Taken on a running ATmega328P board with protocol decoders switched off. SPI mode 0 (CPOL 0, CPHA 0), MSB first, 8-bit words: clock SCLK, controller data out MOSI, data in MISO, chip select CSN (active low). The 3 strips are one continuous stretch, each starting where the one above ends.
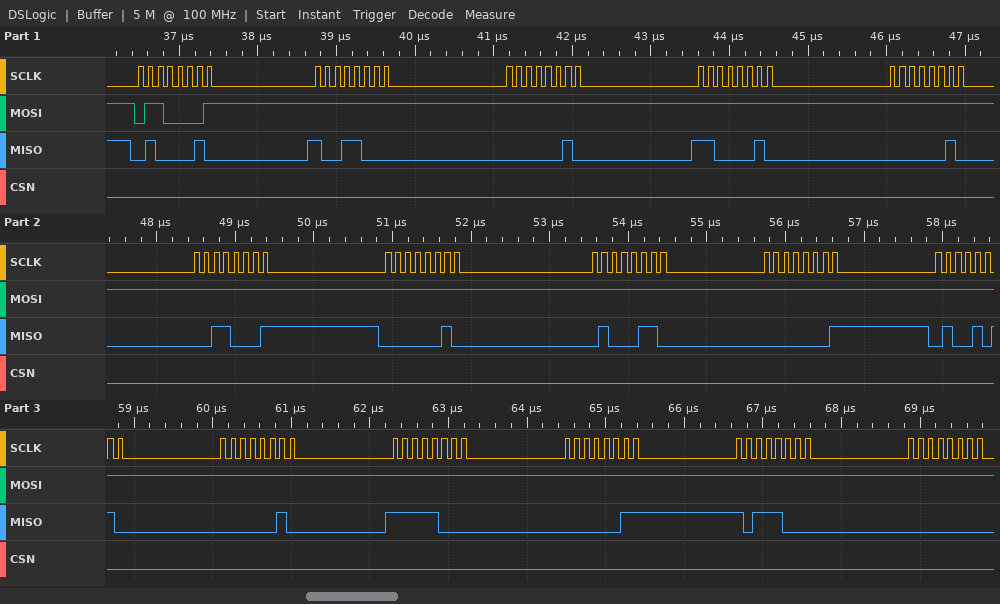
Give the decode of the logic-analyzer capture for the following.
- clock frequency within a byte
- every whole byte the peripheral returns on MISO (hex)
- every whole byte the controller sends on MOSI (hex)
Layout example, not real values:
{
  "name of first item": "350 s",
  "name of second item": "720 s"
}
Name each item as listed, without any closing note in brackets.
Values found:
{
  "clock frequency within a byte": "8 MHz",
  "every whole byte the peripheral returns on MISO": "0x42 0x98 0x02 0xC2 0x02 0x31 0x02 0x46 0x01 0x4A 0x02 0xF8 0x03 0xB8 0x00",
  "every whole byte the controller sends on MOSI": "0x61 0xFF 0xFF 0xFF 0xFF 0xFF 0xFF 0xFF 0xFF 0xFF 0xFF 0xFF 0xFF 0xFF 0xFF"
}
